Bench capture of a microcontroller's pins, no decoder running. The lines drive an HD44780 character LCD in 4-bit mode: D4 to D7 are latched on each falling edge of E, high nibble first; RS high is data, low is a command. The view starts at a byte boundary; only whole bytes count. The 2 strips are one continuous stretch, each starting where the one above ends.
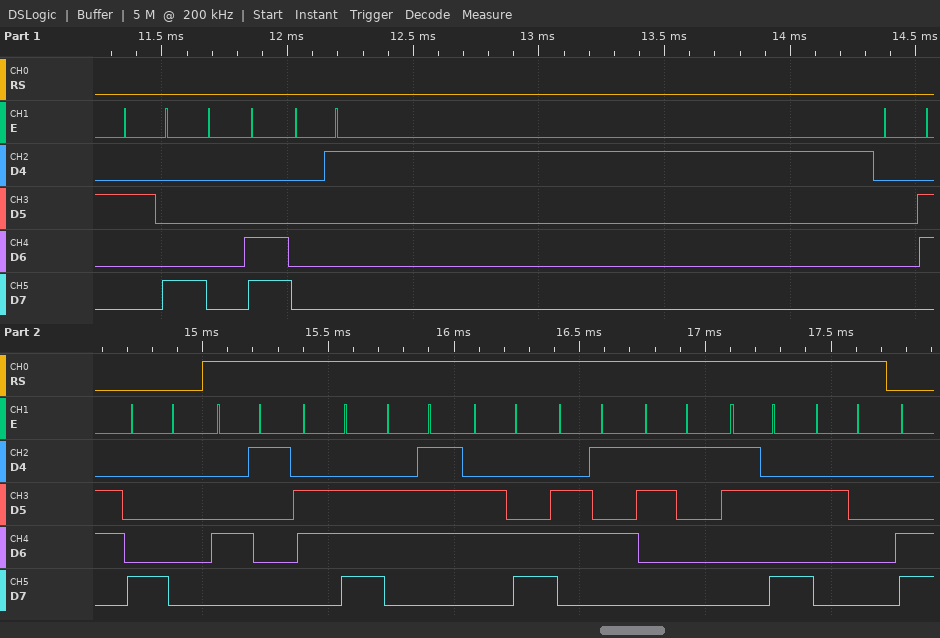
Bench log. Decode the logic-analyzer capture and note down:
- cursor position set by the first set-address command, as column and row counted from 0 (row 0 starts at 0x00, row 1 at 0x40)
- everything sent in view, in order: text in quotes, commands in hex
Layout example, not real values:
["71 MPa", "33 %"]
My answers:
["column 0, row 0", "0x28 0x0C 0x01 0x06 0x80 \"Angle1: \""]
